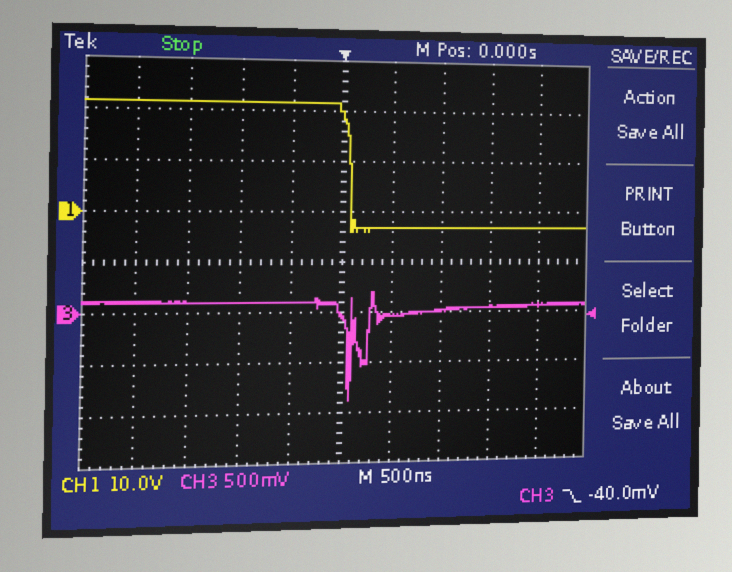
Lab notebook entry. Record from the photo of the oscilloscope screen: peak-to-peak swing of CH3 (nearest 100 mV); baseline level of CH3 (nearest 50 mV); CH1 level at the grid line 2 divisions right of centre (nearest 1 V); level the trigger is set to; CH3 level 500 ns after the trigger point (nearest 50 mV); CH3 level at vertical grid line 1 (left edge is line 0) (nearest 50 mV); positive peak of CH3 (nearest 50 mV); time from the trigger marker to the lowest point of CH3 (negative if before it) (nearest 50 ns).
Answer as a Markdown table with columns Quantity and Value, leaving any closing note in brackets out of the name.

| Quantity | Value |
|---|---|
| peak-to-peak swing of CH3 | 1.10 V |
| baseline level of CH3 | 100 mV |
| CH1 level at the grid line 2 divisions right of centre | -3 V |
| level the trigger is set to | -40.0 mV |
| CH3 level 500 ns after the trigger point | -50 mV |
| CH3 level at vertical grid line 1 (left edge is line 0) | 100 mV |
| positive peak of CH3 | 200 mV |
| time from the trigger marker to the lowest point of CH3 (negative if before it) | +100 ns |
